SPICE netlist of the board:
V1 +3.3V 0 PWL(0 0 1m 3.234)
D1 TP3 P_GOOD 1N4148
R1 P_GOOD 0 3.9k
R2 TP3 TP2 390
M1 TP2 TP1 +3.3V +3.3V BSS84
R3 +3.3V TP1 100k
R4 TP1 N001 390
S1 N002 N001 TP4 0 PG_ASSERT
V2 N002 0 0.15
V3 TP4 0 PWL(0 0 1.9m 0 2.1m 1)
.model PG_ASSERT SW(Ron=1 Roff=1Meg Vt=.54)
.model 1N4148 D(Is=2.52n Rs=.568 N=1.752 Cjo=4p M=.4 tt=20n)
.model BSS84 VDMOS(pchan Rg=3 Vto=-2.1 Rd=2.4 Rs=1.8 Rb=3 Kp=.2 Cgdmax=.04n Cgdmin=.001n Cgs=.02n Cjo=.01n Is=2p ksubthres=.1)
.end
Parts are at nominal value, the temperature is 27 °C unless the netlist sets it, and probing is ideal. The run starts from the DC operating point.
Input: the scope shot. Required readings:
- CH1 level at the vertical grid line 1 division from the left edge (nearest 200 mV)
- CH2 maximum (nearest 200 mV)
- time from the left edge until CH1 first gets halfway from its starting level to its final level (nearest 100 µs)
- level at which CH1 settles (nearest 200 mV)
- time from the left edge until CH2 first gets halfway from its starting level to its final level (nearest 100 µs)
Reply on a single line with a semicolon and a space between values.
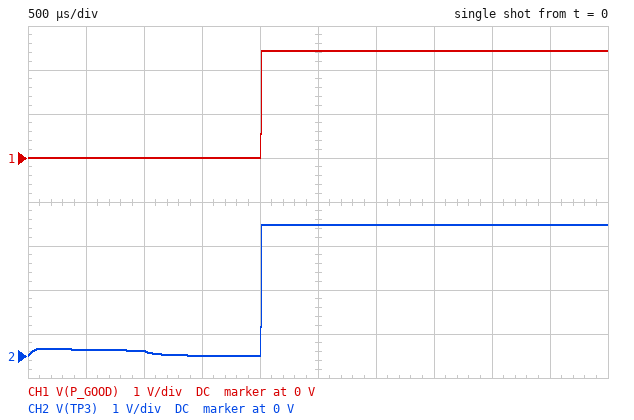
0 V; 3.0 V; 2.0 ms; 2.4 V; 2.0 ms
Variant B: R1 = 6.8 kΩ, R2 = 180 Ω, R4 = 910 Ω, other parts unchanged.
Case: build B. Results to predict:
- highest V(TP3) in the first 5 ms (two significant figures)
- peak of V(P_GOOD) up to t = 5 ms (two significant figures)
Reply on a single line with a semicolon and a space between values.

3.2 V; 2.6 V
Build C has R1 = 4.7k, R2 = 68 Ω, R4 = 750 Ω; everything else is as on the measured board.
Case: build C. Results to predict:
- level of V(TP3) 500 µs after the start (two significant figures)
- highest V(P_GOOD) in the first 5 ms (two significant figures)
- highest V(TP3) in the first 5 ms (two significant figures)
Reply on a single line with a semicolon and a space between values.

140 mV; 2.6 V; 3.2 V
